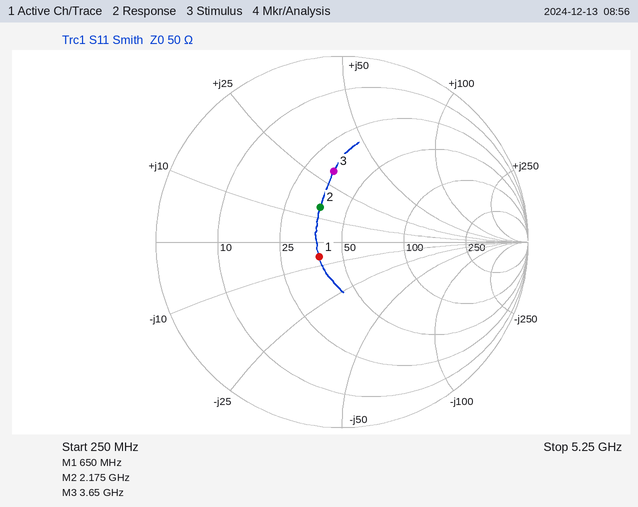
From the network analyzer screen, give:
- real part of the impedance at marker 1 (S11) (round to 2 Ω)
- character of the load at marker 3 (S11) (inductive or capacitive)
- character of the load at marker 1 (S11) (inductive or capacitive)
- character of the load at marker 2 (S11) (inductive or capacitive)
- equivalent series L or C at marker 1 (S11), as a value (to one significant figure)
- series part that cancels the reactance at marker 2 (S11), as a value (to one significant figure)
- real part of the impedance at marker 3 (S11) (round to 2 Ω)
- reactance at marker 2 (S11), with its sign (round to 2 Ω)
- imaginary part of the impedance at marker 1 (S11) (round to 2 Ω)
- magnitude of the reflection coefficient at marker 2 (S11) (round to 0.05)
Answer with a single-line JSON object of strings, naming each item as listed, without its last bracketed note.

{"real part of the impedance at marker 1 (S11)": "38 Ω", "character of the load at marker 3 (S11)": "inductive", "character of the load at marker 1 (S11)": "capacitive", "character of the load at marker 2 (S11)": "inductive", "equivalent series L or C at marker 1 (S11), as a value": "40 pF", "series part that cancels the reactance at marker 2 (S11), as a value": "5 pF", "real part of the impedance at marker 3 (S11)": "34 Ω", "reactance at marker 2 (S11), with its sign": "+14 Ω", "imaginary part of the impedance at marker 1 (S11)": "-6 Ω", "magnitude of the reflection coefficient at marker 2 (S11)": "0.20"}
